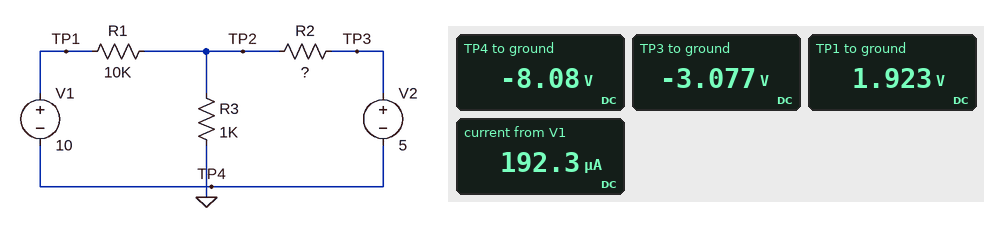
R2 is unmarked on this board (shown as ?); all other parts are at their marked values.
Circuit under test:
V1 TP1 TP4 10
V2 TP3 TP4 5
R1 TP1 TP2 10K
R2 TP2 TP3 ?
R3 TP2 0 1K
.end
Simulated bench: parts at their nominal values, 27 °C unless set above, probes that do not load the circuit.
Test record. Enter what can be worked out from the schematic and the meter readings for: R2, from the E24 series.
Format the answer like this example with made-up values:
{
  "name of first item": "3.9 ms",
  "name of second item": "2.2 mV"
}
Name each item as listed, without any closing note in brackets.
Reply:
{
  "R2, from the E24 series": "16 kΩ"
}
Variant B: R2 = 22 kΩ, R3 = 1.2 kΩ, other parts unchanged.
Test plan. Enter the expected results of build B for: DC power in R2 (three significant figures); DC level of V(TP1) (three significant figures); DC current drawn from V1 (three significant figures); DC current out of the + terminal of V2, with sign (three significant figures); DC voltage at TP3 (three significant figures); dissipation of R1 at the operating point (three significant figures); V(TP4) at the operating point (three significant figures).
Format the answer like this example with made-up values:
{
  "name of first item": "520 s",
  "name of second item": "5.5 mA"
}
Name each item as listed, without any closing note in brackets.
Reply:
{
  "DC power in R2": "537 µW",
  "DC level of V(TP1)": "1.56 V",
  "DC current drawn from V1": "156 µA",
  "DC current out of the + terminal of V2, with sign": "-156 µA",
  "DC voltage at TP3": "-3.44 V",
  "dissipation of R1 at the operating point": "244 µW",
  "V(TP4) at the operating point": "-8.44 V"
}
